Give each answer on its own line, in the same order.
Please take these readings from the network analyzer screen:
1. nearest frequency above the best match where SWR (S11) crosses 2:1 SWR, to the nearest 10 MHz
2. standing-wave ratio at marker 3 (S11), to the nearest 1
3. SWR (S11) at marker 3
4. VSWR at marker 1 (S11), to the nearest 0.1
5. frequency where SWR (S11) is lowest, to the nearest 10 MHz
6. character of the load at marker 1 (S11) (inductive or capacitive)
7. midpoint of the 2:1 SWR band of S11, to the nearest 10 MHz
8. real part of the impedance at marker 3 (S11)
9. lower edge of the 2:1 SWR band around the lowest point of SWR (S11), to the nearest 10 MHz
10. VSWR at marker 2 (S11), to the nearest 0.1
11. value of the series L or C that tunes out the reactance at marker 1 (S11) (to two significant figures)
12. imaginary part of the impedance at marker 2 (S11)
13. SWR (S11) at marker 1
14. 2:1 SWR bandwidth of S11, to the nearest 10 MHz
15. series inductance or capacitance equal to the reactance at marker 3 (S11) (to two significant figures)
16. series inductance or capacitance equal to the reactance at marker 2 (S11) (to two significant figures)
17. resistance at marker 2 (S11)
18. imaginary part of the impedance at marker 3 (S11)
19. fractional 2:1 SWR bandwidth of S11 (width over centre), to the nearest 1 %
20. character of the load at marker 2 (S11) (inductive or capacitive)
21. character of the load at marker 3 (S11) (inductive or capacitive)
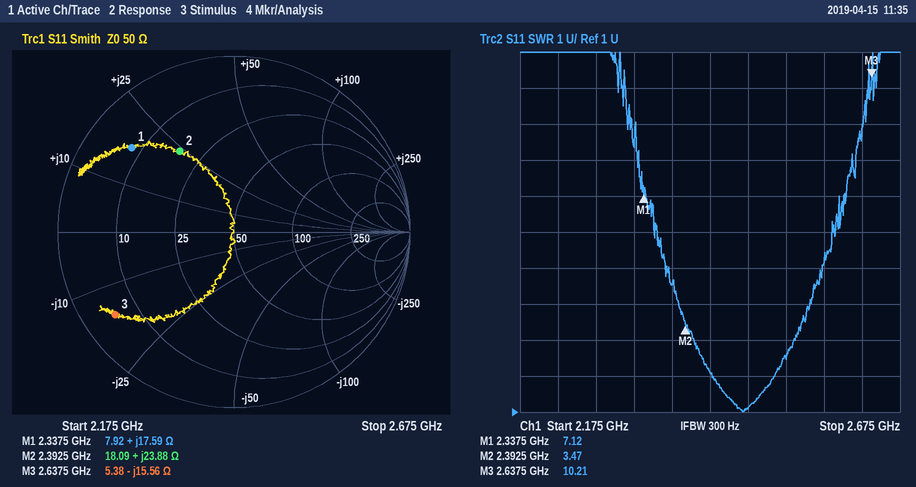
2.51 GHz
10
10.21
7.1
2.47 GHz
inductive
2.47 GHz
5.38 Ω
2.43 GHz
3.5
3.9 pF
+23.88 Ω
7.12
80 MHz
3.9 pF
1.6 nH
18.09 Ω
-15.56 Ω
3 %
inductive
capacitive
